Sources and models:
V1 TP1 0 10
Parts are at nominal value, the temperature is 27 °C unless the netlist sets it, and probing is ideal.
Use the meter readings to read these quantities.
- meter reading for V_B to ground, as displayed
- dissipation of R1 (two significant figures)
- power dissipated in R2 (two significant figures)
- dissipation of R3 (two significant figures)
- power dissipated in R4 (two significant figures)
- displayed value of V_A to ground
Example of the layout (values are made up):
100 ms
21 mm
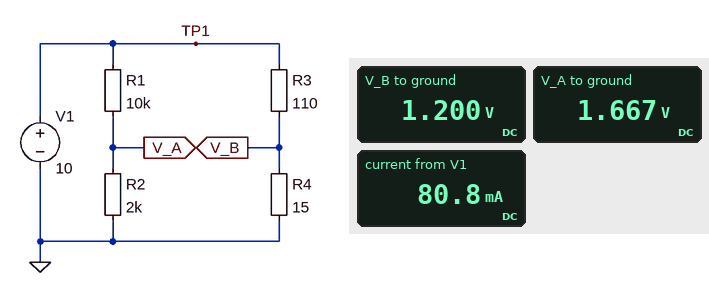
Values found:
1.200 V
6.9 mW
1.4 mW
700 mW
96 mW
1.667 V
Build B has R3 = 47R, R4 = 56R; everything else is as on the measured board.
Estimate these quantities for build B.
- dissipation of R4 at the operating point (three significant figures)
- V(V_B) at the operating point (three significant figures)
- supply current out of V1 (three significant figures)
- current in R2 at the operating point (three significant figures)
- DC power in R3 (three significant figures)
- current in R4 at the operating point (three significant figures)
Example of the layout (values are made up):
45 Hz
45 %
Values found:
528 mW
5.44 V
97.9 mA
833 µA
443 mW
97.1 mA
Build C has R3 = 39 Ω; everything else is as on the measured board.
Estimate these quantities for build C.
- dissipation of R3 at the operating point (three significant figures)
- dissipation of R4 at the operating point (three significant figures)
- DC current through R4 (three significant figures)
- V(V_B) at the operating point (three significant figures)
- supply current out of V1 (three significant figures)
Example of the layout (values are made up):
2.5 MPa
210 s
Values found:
1.34 W
514 mW
185 mA
2.78 V
186 mA
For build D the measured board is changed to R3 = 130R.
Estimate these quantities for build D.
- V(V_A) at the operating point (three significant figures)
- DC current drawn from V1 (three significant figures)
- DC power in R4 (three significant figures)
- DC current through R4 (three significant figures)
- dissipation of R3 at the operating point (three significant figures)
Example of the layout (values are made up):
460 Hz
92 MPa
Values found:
1.67 V
69.8 mA
71.3 mW
69.0 mA
618 mW
